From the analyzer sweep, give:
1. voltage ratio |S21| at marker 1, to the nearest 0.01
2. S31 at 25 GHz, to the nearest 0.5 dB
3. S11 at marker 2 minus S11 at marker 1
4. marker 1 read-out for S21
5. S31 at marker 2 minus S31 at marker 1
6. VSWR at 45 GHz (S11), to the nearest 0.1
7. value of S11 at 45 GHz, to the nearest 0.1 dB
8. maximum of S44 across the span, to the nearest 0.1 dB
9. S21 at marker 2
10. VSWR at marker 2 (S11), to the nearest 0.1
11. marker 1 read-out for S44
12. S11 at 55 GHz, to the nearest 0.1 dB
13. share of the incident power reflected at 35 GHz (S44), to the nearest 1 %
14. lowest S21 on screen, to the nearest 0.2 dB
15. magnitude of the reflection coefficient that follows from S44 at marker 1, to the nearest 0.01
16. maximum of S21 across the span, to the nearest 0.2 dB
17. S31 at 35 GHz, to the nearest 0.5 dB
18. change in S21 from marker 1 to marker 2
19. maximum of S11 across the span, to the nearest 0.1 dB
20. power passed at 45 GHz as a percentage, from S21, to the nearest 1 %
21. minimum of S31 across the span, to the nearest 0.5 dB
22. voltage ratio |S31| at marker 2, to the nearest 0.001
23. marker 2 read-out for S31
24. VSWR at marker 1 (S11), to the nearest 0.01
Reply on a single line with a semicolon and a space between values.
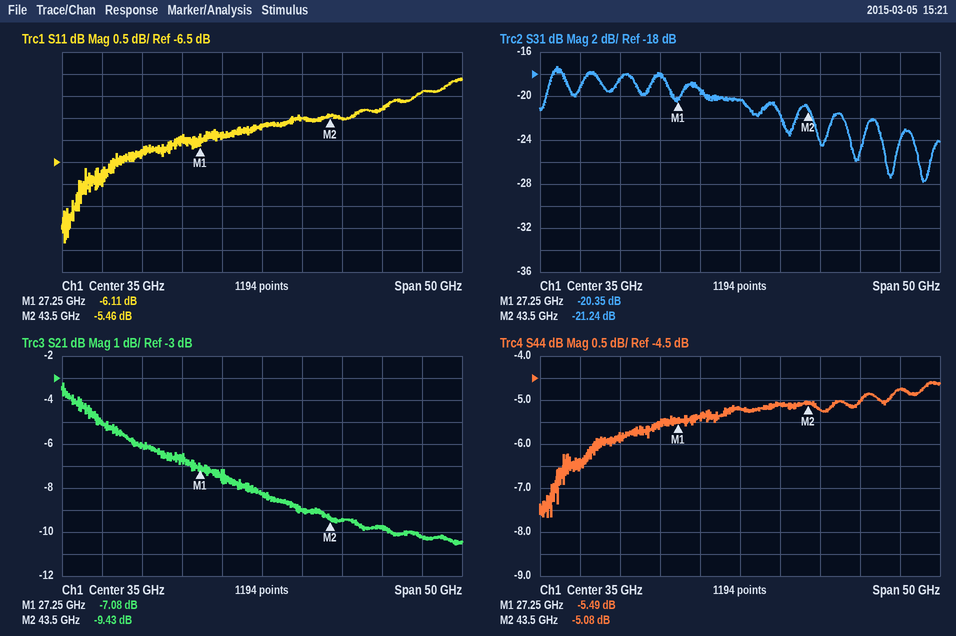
0.44; -18.0 dB; 0.65 dB; -7.08 dB; -0.89 dB; 3.3; -5.5 dB; -4.6 dB; -9.43 dB; 3.3; -5.49 dB; -4.9 dB; 30 %; -10.6 dB; 0.53; -3.2 dB; -20.5 dB; -2.35 dB; -4.6 dB; 11 %; -28.0 dB; 0.087; -21.24 dB; 2.96
